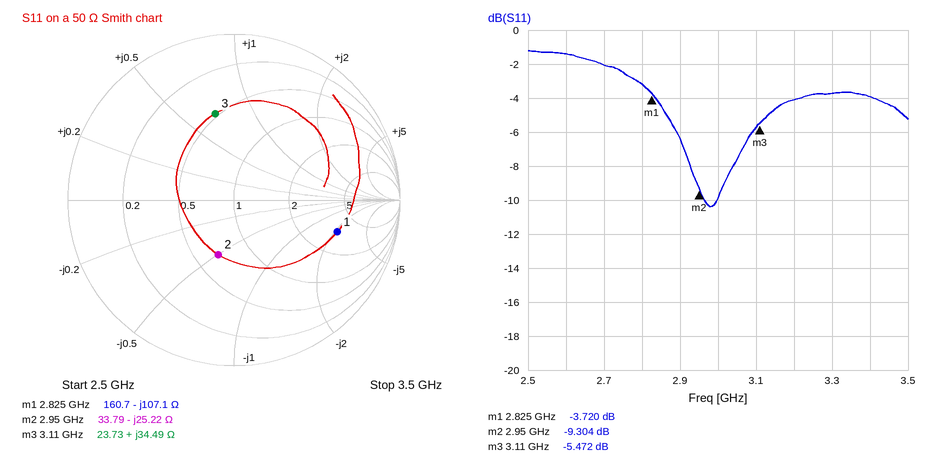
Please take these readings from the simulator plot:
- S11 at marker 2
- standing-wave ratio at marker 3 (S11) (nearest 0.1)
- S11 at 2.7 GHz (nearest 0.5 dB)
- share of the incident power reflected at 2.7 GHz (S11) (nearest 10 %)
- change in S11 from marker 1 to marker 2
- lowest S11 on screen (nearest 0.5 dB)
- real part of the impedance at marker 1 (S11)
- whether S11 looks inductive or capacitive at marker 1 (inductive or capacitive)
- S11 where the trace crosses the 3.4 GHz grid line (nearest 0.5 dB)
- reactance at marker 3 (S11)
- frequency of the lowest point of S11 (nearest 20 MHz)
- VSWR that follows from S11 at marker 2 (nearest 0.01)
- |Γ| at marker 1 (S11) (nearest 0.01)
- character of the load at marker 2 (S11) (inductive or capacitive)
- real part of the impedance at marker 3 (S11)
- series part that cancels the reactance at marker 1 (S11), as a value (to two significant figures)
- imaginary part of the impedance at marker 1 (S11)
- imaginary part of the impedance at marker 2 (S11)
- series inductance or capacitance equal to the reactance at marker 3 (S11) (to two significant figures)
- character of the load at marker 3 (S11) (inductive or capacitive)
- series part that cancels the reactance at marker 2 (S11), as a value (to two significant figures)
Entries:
-9.304 dB
3.3
-2.0 dB
60 %
-5.584 dB
-10.5 dB
160.7 Ω
capacitive
-4.0 dB
+34.49 Ω
2.98 GHz
2.04
0.65
capacitive
23.73 Ω
6.0 nH
-107.1 Ω
-25.22 Ω
1.8 nH
inductive
1.4 nH
